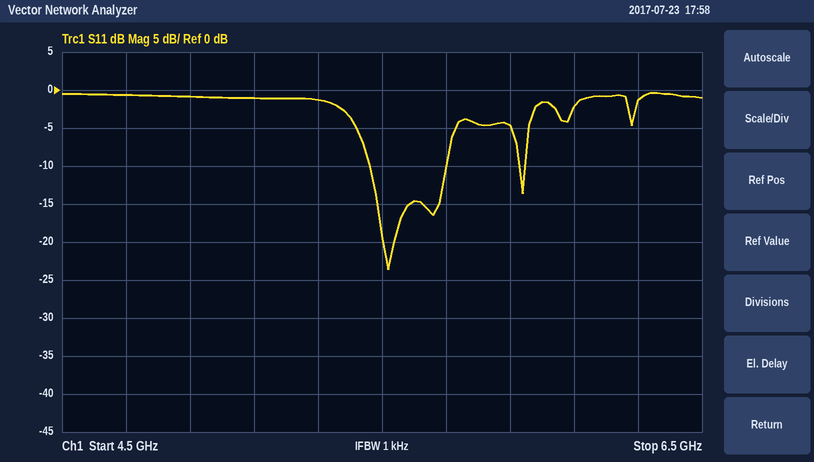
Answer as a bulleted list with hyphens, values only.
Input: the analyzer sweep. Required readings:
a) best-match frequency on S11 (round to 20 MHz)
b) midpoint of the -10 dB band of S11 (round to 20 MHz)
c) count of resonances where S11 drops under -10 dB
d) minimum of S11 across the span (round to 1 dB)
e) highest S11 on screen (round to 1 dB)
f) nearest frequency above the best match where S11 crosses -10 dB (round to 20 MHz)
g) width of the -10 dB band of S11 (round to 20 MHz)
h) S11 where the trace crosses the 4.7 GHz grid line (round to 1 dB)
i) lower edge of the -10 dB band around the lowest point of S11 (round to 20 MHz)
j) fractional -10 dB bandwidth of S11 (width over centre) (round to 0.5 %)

- 5.52 GHz
- 5.58 GHz
- 2
- -24 dB
- 0 dB
- 5.70 GHz
- 240 MHz
- -1 dB
- 5.46 GHz
- 4.5 %
